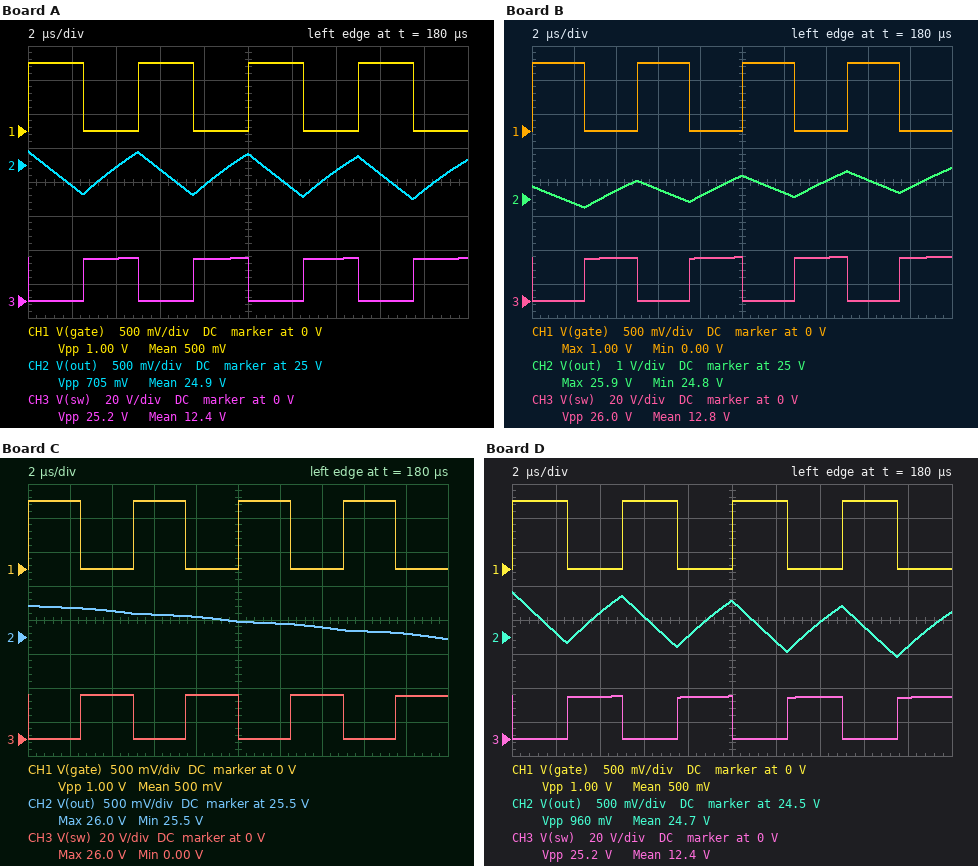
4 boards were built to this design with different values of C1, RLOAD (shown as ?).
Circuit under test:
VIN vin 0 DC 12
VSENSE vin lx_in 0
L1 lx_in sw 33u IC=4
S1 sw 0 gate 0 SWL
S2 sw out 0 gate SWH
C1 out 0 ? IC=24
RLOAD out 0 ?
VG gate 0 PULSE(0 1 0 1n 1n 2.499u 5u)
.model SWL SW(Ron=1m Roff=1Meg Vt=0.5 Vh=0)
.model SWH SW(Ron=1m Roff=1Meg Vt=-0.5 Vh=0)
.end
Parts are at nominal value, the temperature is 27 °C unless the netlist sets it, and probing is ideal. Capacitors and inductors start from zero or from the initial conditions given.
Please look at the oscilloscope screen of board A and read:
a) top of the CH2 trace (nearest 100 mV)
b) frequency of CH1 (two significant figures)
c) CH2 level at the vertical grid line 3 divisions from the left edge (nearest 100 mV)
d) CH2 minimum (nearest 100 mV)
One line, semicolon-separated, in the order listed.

25.2 V; 200 kHz; 24.9 V; 24.5 V
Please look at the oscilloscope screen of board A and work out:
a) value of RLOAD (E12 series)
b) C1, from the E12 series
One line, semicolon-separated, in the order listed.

8.2 Ω; 12 µF
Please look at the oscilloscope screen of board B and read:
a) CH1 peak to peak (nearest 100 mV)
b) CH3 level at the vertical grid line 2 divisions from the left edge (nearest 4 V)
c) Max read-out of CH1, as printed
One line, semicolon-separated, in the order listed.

1.0 V; 24 V; 1.00 V
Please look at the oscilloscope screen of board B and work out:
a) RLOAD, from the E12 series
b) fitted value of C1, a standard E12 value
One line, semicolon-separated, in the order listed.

5.6 Ω; 18 µF
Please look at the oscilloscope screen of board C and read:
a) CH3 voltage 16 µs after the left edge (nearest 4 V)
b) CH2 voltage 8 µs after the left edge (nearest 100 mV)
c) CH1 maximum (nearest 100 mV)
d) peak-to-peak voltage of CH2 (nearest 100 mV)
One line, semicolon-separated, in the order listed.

0 V; 25.8 V; 1.0 V; 500 mV
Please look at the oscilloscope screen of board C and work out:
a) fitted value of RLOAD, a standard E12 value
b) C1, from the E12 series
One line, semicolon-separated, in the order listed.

39 Ω; 47 µF
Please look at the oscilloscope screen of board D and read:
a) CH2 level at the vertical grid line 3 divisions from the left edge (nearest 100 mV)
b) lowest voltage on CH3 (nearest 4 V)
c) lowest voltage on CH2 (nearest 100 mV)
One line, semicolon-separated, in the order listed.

24.8 V; 0 V; 24.2 V
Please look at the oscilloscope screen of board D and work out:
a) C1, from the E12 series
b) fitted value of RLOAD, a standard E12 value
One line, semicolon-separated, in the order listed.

10 µF; 8.2 Ω
